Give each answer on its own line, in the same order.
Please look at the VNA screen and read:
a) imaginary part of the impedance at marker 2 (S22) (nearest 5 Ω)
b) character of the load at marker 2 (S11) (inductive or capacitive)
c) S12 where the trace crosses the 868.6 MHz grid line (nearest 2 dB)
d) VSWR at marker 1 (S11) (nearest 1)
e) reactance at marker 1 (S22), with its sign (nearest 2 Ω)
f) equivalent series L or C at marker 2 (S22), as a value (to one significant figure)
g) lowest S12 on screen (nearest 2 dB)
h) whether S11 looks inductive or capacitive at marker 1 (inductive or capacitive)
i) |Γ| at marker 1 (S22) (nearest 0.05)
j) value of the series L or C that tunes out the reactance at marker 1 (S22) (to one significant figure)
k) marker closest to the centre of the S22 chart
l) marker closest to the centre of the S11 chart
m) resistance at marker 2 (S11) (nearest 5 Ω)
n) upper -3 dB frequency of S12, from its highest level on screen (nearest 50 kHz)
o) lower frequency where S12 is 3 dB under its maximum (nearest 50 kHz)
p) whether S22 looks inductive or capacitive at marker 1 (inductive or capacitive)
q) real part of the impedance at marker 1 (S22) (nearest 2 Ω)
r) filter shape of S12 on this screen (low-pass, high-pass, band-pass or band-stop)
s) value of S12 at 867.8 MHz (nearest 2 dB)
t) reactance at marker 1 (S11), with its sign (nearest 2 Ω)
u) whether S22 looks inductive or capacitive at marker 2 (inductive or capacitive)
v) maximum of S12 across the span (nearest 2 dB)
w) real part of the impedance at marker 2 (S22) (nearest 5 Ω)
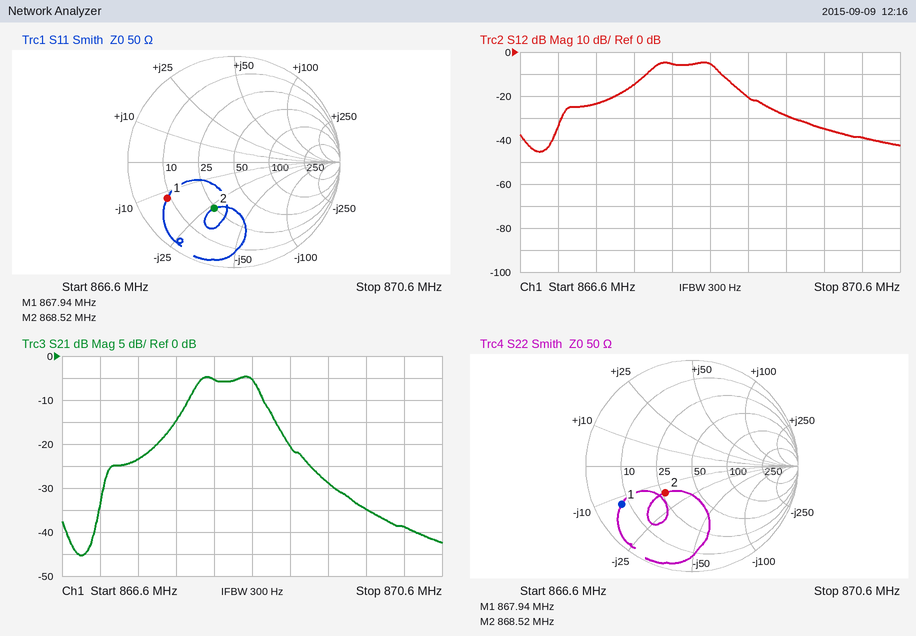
-15 Ω
capacitive
-6 dB
6
-12 Ω
10 pF
-46 dB
capacitive
0.75
2 nH
marker 2
marker 2
25 Ω
868.65 MHz
868.00 MHz
capacitive
8 Ω
band-pass
-14 dB
-12 Ω
capacitive
-4 dB
25 Ω
